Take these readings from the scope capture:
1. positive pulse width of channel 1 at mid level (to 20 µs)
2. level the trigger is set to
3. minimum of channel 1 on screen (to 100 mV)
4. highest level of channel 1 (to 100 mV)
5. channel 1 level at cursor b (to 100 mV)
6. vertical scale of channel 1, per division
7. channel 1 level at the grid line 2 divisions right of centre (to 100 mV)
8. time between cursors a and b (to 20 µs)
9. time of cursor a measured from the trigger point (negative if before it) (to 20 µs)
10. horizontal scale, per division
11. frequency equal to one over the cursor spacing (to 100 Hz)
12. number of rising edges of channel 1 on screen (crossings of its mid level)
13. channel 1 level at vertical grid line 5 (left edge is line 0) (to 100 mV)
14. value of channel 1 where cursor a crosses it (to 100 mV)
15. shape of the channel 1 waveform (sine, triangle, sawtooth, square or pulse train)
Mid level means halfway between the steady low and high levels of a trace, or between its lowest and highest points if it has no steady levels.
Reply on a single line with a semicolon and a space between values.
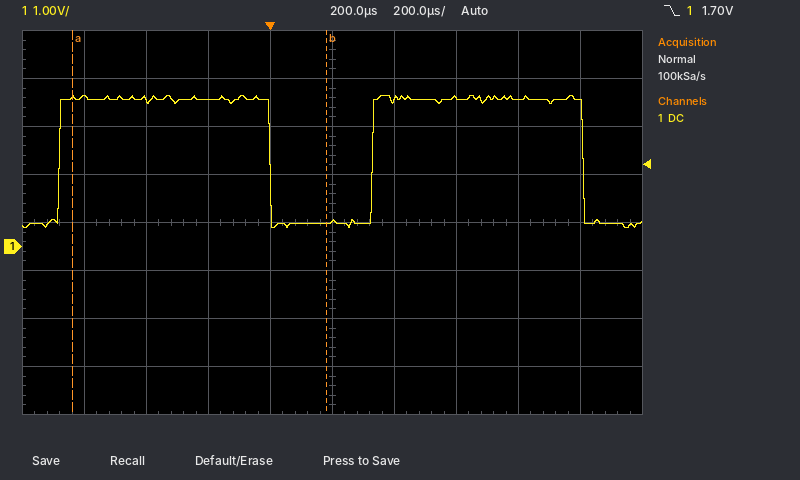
680 µs; 1.70 V; 400 mV; 3.1 V; 500 mV; 1 V; 3.1 V; 820 µs; -640 µs; 200 µs; 1.2 kHz; 2; 500 mV; 3.1 V; pulse train
